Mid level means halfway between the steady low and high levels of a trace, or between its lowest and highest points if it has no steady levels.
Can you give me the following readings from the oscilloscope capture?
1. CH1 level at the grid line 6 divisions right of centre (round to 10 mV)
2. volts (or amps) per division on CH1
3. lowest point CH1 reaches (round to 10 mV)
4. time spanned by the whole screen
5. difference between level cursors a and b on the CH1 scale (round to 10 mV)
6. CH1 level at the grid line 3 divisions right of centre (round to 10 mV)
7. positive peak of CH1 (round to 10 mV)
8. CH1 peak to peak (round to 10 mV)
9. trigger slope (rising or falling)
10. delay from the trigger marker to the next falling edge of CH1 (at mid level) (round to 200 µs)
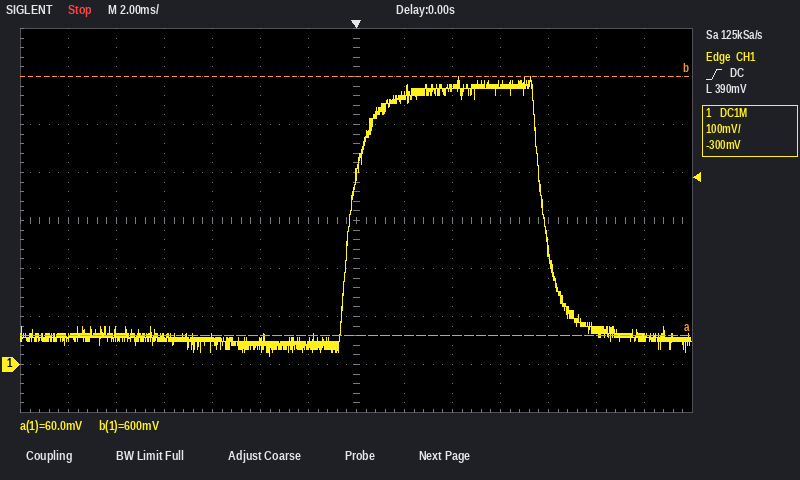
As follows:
60 mV
100 mV
20 mV
28 ms
540 mV
580 mV
600 mV
580 mV
rising
7.8 ms
